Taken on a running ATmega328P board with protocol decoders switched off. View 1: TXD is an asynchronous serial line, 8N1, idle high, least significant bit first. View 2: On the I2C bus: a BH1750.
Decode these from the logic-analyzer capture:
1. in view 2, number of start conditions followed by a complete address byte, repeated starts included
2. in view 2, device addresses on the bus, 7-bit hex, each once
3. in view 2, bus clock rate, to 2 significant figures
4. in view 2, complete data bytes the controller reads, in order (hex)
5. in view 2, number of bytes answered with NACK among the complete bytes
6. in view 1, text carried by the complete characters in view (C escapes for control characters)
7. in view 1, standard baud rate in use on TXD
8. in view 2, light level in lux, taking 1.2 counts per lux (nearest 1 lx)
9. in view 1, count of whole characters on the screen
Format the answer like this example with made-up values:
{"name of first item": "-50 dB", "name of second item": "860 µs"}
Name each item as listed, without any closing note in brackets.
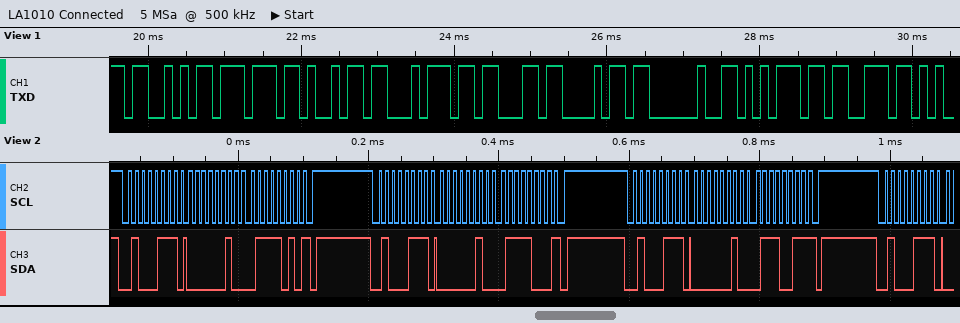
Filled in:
{"in view 2, number of start conditions followed by a complete address byte, repeated starts included": "4", "in view 2, device addresses on the bus, 7-bit hex, each once": "0x23", "in view 2, bus clock rate, to 2 significant figures": "100 kHz", "in view 2, complete data bytes the controller reads, in order": "02 7A 02 78 02 73", "in view 2, number of bytes answered with NACK among the complete bytes": "3", "in view 1, text carried by the complete characters in view": "\"Switch us\"", "in view 1, standard baud rate in use on TXD": "9600 baud", "in view 2, light level in lux, taking 1.2 counts per lux": "528 lx", "in view 1, count of whole characters on the screen": "9"}
